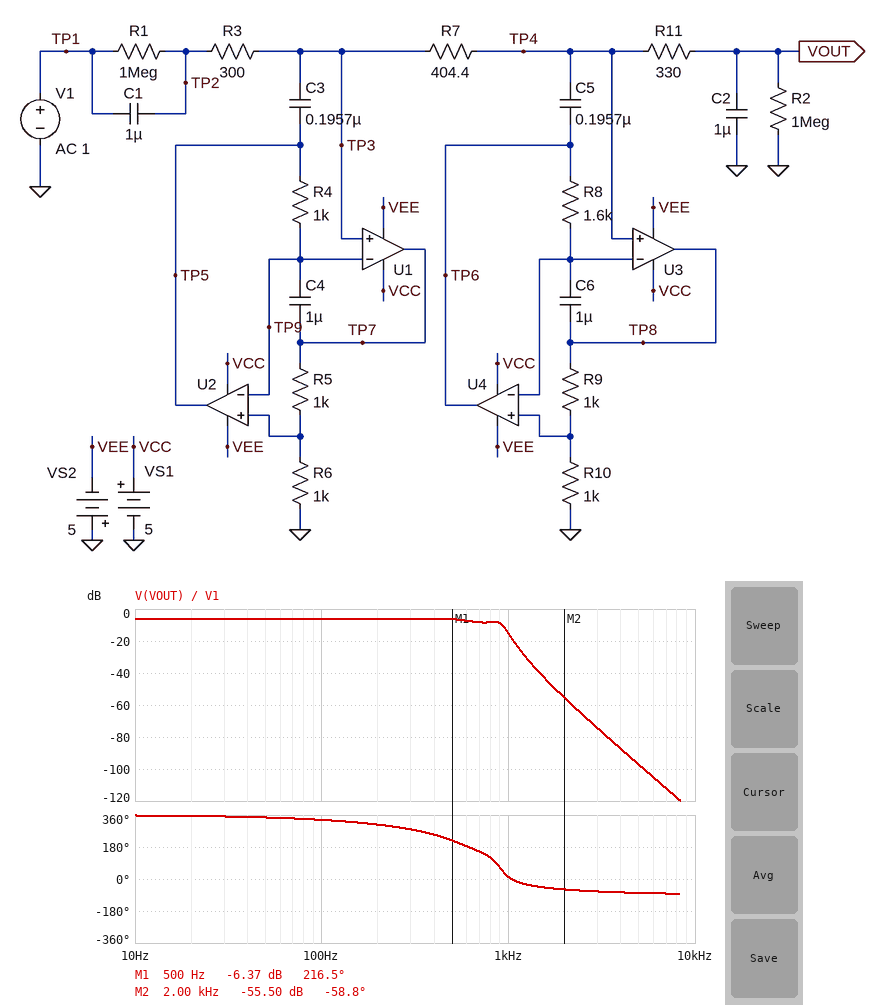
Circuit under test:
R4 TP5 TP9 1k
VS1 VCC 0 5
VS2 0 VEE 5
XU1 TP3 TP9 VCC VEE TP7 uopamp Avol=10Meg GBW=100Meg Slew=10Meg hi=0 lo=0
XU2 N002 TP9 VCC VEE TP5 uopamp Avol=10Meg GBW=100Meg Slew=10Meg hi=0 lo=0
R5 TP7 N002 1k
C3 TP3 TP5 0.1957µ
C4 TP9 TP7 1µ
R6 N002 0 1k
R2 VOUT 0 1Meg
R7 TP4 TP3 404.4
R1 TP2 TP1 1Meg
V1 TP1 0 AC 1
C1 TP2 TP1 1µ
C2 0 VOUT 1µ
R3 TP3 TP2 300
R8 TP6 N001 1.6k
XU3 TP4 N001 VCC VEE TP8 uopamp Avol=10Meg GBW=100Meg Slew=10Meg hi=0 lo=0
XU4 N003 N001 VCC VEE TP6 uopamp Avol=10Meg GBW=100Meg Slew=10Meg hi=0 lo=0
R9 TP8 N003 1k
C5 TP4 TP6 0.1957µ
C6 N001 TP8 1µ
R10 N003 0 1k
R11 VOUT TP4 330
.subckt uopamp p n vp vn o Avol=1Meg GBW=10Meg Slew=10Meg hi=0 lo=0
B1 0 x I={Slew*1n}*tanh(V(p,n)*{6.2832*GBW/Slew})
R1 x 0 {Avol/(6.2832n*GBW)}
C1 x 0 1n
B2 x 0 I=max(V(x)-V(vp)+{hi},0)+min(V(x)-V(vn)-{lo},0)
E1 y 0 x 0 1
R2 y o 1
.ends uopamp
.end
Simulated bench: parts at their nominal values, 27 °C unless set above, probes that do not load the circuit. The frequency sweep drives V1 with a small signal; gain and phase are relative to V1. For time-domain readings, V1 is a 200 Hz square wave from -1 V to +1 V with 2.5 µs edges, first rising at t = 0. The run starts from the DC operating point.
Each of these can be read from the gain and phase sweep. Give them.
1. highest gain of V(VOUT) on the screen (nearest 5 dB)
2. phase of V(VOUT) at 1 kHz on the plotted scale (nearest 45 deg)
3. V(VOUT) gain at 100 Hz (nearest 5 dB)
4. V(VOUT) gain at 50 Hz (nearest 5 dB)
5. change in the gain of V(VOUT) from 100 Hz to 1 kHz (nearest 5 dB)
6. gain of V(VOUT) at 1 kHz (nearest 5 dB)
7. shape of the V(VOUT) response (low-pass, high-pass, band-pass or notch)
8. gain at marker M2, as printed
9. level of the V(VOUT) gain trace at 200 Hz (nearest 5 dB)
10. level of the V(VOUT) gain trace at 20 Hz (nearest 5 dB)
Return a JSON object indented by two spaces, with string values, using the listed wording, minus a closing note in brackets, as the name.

{
  "highest gain of V(VOUT) on the screen": "-5 dB",
  "phase of V(VOUT) at 1 kHz on the plotted scale": "0 deg",
  "V(VOUT) gain at 100 Hz": "-5 dB",
  "V(VOUT) gain at 50 Hz": "-5 dB",
  "change in the gain of V(VOUT) from 100 Hz to 1 kHz": "-10 dB",
  "gain of V(VOUT) at 1 kHz": "-15 dB",
  "shape of the V(VOUT) response": "low-pass",
  "gain at marker M2, as printed": "-55.50 dB",
  "level of the V(VOUT) gain trace at 200 Hz": "-5 dB",
  "level of the V(VOUT) gain trace at 20 Hz": "-5 dB"
}
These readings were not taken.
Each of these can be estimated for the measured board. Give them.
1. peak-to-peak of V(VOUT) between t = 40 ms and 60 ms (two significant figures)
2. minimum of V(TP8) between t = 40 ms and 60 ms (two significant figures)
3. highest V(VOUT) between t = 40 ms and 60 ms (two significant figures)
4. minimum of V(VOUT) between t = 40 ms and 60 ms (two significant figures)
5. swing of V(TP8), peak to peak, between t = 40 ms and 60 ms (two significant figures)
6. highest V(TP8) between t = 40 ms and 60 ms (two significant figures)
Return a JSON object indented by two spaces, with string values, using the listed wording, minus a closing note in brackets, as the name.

{
  "peak-to-peak of V(VOUT) between t = 40 ms and 60 ms": "1.2 V",
  "minimum of V(TP8) between t = 40 ms and 60 ms": "-1.7 V",
  "highest V(VOUT) between t = 40 ms and 60 ms": "620 mV",
  "minimum of V(VOUT) between t = 40 ms and 60 ms": "-620 mV",
  "swing of V(TP8), peak to peak, between t = 40 ms and 60 ms": "3.4 V",
  "highest V(TP8) between t = 40 ms and 60 ms": "1.7 V"
}
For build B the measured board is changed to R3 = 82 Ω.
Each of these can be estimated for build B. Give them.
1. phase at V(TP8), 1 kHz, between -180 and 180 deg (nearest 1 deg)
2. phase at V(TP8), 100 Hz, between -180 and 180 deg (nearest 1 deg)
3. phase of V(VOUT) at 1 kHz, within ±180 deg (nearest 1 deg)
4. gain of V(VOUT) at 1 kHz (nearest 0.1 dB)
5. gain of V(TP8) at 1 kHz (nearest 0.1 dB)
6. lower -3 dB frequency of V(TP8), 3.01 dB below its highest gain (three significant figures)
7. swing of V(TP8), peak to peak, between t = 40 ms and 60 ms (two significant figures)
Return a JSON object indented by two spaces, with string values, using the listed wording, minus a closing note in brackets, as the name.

{
  "phase at V(TP8), 1 kHz, between -180 and 180 deg": "141 deg",
  "phase at V(TP8), 100 Hz, between -180 and 180 deg": "-12 deg",
  "phase of V(VOUT) at 1 kHz, within ±180 deg": "77 deg",
  "gain of V(VOUT) at 1 kHz": "-16.7 dB",
  "gain of V(TP8) at 1 kHz": "-3.4 dB",
  "lower -3 dB frequency of V(TP8), 3.01 dB below its highest gain": "273 Hz",
  "swing of V(TP8), peak to peak, between t = 40 ms and 60 ms": "3.3 V"
}
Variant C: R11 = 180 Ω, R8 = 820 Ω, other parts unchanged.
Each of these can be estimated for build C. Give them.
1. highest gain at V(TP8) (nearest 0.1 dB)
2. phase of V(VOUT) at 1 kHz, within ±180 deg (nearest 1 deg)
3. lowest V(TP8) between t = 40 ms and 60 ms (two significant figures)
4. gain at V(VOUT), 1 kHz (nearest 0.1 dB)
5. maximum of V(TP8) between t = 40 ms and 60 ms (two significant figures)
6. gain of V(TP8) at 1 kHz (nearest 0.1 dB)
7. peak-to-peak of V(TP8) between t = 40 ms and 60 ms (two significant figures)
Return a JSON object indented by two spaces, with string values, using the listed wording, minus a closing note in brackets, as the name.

{
  "highest gain at V(TP8)": "2.3 dB",
  "phase of V(VOUT) at 1 kHz, within ±180 deg": "113 deg",
  "lowest V(TP8) between t = 40 ms and 60 ms": "-1.5 V",
  "gain at V(VOUT), 1 kHz": "-7.6 dB",
  "maximum of V(TP8) between t = 40 ms and 60 ms": "1.5 V",
  "gain of V(TP8) at 1 kHz": "2.0 dB",
  "peak-to-peak of V(TP8) between t = 40 ms and 60 ms": "3.0 V"
}
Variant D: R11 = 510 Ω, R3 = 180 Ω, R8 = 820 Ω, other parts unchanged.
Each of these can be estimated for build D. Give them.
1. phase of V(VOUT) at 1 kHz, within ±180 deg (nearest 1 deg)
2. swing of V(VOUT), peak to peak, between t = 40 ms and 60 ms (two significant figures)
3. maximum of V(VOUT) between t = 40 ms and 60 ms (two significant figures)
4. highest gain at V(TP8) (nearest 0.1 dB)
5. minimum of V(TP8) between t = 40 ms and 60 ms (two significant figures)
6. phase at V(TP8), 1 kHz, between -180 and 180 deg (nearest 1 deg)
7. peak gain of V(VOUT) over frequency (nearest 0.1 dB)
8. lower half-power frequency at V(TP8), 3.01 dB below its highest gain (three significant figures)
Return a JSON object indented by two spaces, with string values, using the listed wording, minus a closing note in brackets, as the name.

{
  "phase of V(VOUT) at 1 kHz, within ±180 deg": "84 deg",
  "swing of V(VOUT), peak to peak, between t = 40 ms and 60 ms": "1.1 V",
  "maximum of V(VOUT) between t = 40 ms and 60 ms": "570 mV",
  "highest gain at V(TP8)": "8.8 dB",
  "minimum of V(TP8) between t = 40 ms and 60 ms": "-2.4 V",
  "phase at V(TP8), 1 kHz, between -180 and 180 deg": "156 deg",
  "peak gain of V(VOUT) over frequency": "-6.0 dB",
  "lower half-power frequency at V(TP8), 3.01 dB below its highest gain": "605 Hz"
}
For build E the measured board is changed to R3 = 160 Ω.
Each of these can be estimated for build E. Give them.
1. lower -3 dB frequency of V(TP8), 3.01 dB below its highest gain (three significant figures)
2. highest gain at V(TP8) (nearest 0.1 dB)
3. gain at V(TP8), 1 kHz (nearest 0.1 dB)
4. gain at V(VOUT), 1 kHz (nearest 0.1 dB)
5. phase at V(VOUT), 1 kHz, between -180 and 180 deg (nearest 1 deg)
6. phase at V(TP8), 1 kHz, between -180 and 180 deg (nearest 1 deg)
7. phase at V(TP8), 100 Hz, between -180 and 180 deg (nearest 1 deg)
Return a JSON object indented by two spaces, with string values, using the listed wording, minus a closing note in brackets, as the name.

{
  "lower -3 dB frequency of V(TP8), 3.01 dB below its highest gain": "216 Hz",
  "highest gain at V(TP8)": "3.6 dB",
  "gain at V(TP8), 1 kHz": "-1.6 dB",
  "gain at V(VOUT), 1 kHz": "-14.9 dB",
  "phase at V(VOUT), 1 kHz, between -180 and 180 deg": "58 deg",
  "phase at V(TP8), 1 kHz, between -180 and 180 deg": "122 deg",
  "phase at V(TP8), 100 Hz, between -180 and 180 deg": "-13 deg"
}
